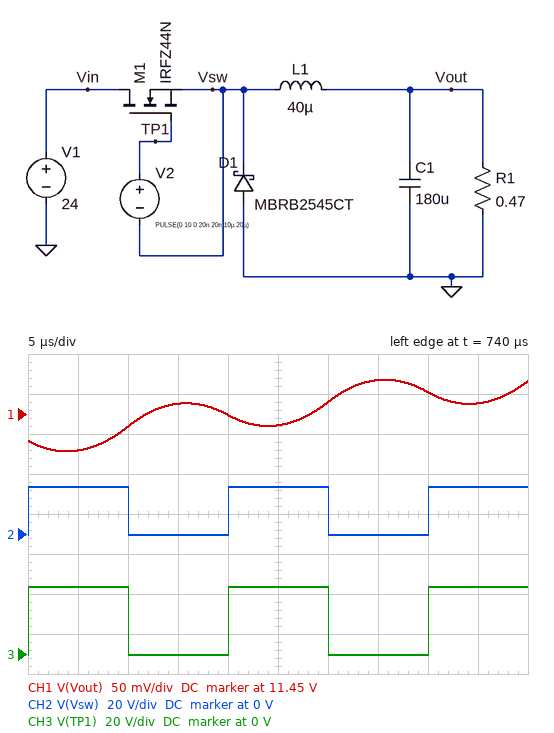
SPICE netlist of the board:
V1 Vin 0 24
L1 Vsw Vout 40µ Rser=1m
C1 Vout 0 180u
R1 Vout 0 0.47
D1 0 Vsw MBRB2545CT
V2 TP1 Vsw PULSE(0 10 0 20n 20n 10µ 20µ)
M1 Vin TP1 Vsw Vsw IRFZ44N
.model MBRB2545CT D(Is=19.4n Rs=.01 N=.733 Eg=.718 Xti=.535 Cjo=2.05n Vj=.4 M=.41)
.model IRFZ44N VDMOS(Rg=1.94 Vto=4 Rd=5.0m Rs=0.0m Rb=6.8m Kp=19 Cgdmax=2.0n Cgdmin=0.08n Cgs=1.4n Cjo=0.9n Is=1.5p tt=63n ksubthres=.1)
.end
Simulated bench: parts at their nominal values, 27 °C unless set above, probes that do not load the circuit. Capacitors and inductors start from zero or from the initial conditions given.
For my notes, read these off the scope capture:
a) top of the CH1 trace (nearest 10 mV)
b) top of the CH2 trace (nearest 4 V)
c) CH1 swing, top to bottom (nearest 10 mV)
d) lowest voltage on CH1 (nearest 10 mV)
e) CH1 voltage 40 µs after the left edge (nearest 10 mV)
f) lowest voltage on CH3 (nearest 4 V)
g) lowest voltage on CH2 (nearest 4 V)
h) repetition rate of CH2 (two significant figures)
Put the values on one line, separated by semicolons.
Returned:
11.49 V; 24 V; 90 mV; 11.40 V; 11.48 V; 0 V; 0 V; 50 kHz
